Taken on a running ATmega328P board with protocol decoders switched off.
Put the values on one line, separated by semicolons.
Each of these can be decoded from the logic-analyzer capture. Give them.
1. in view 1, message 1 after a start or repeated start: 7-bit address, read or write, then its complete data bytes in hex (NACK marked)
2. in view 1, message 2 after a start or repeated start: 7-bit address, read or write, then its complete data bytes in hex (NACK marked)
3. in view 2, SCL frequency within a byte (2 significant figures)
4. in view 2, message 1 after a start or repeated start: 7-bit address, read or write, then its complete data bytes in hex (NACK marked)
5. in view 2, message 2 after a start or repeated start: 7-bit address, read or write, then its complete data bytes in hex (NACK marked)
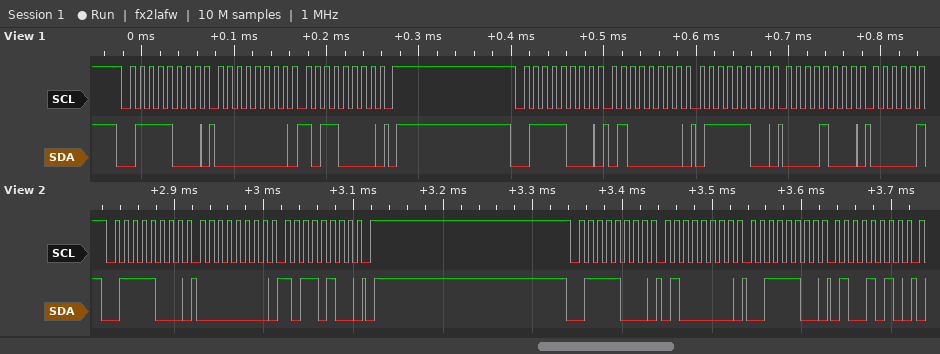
0x3C write: 00 B0; 0x3C write: 40 7C 08; 100 kHz; 0x3C write: 00 B4; 0x3C write: 40 3C 4A
